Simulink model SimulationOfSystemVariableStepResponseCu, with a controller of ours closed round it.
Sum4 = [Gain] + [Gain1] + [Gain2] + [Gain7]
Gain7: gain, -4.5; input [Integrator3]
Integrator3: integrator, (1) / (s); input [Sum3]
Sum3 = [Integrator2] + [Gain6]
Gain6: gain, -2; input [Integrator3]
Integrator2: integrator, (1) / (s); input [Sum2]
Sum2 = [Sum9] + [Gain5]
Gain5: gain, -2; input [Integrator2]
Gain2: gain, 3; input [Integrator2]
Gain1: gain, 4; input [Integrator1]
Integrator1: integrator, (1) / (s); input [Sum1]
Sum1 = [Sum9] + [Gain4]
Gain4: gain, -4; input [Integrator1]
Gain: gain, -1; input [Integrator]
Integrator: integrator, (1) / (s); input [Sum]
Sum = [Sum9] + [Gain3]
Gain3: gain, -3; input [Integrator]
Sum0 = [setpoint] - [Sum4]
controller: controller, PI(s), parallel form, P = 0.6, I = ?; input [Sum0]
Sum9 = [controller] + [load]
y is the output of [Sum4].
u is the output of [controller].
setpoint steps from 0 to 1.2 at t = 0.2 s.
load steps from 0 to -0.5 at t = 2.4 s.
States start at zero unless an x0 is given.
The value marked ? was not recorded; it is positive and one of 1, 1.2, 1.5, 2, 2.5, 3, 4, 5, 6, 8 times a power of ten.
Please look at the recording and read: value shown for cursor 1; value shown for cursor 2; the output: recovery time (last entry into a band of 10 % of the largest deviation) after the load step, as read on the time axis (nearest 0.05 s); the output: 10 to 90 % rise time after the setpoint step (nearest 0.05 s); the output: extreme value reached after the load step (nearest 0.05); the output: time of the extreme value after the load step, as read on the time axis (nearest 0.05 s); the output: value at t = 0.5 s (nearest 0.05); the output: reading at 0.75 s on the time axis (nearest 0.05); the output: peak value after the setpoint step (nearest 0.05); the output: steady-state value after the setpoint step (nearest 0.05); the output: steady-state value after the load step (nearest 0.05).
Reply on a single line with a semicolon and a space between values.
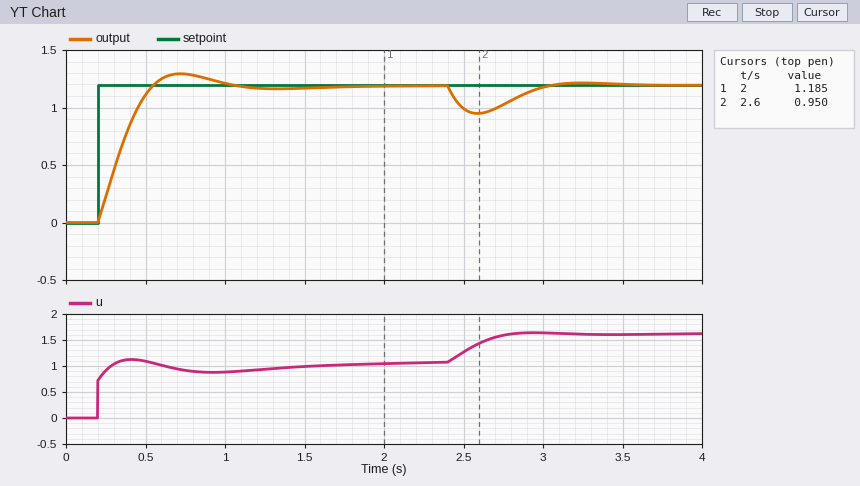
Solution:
1.185; 0.950; 3.00 s; 0.25 s; 0.95; 2.60 s; 1.10; 1.30; 1.30; 1.20; 1.20
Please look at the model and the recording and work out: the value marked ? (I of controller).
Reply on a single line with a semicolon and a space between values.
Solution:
6
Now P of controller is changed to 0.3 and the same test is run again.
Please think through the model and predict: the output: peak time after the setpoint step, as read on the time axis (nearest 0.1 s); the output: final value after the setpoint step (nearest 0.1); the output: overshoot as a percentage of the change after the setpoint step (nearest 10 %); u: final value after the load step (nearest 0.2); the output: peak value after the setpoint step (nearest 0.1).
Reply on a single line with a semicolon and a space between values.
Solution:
0.7 s; 1.2; 20 %; 1.6; 1.4
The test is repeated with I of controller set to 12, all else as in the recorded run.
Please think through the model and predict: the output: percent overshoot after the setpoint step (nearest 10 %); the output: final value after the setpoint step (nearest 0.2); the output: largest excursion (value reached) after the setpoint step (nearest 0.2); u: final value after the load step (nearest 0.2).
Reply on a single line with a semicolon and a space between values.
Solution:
20 %; 1.2; 1.4; 1.6
